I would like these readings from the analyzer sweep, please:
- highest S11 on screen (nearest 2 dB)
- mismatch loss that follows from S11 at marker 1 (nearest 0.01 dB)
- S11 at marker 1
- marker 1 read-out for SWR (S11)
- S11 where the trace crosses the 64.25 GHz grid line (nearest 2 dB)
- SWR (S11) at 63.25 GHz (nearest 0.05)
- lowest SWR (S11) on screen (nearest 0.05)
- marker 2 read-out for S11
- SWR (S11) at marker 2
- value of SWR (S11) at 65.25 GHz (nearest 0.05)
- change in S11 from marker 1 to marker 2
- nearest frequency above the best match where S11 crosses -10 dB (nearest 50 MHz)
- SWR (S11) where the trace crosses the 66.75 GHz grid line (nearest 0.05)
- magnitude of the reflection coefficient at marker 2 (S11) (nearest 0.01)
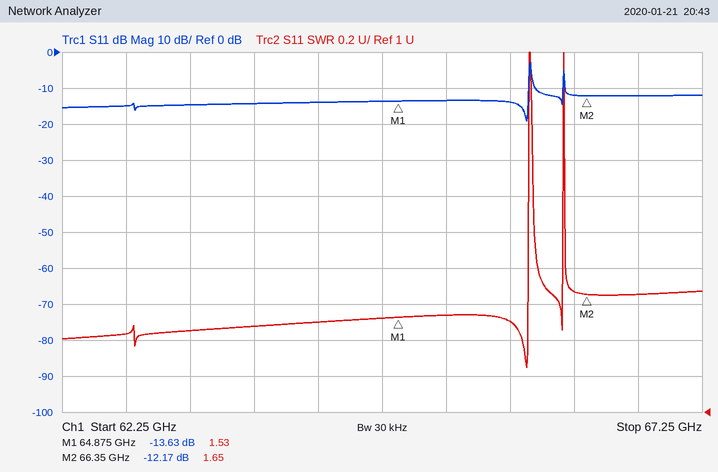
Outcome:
-2 dB
0.19 dB
-13.63 dB
1.53
-14 dB
1.45
1.25
-12.17 dB
1.65
1.55
1.46 dB
65.90 GHz
1.65
0.25
